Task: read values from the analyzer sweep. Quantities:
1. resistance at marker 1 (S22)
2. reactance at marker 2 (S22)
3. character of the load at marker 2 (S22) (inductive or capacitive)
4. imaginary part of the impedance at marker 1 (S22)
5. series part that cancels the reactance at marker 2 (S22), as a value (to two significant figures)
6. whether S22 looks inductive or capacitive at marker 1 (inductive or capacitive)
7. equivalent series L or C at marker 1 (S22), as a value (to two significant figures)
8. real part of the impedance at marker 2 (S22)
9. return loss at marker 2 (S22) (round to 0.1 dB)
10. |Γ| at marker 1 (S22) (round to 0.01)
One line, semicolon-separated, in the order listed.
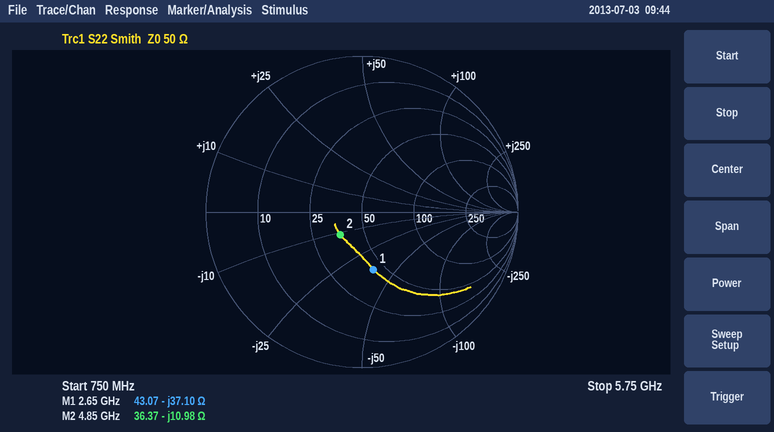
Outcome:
43.07 Ω; -10.98 Ω; capacitive; -37.10 Ω; 360 pH; capacitive; 1.6 pF; 36.37 Ω; 13.9 dB; 0.38
